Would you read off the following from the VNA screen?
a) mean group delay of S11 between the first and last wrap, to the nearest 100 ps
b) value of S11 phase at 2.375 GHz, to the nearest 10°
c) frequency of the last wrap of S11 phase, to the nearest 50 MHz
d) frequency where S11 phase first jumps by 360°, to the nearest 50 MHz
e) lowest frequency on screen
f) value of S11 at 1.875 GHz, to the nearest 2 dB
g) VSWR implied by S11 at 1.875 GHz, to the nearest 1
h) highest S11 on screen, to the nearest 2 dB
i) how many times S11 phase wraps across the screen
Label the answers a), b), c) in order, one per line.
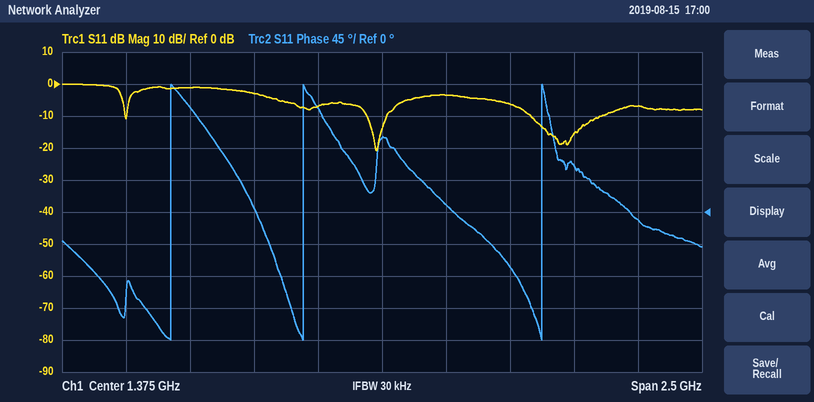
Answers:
a) 1.4 ns
b) -10°
c) 2.00 GHz
d) 550 MHz
e) 125 MHz
f) -6 dB
g) 3
h) 0 dB
i) 3
